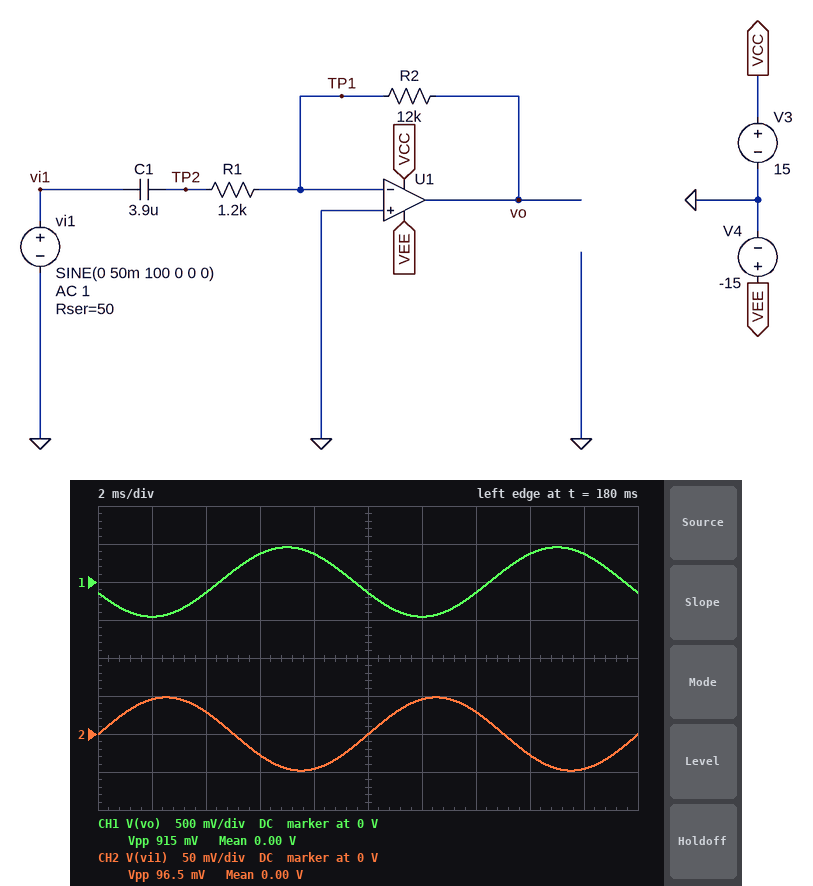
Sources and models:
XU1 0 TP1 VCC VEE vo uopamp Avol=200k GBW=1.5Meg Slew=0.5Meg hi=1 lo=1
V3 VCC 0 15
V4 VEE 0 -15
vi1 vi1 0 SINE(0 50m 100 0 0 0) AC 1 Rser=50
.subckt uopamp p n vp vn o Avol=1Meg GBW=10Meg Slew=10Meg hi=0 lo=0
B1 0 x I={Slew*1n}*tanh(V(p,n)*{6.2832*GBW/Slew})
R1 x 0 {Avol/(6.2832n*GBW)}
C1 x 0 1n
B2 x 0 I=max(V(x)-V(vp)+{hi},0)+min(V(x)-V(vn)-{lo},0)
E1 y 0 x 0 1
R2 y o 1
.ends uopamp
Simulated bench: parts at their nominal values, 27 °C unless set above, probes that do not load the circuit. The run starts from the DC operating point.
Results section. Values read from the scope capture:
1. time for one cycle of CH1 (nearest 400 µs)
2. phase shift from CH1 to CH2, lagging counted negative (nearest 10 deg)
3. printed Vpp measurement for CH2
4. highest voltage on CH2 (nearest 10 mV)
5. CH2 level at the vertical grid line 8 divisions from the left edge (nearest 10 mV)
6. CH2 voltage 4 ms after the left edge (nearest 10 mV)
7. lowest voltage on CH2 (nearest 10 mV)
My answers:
10.0 ms
160 deg
96.5 mV
50 mV
-30 mV
30 mV
-50 mV
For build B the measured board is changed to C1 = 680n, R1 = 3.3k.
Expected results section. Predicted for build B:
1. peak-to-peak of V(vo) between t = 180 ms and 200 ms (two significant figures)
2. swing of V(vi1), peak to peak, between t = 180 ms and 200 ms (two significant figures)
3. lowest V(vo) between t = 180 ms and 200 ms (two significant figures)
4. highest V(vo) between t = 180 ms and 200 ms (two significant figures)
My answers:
290 mV
99 mV
-150 mV
150 mV
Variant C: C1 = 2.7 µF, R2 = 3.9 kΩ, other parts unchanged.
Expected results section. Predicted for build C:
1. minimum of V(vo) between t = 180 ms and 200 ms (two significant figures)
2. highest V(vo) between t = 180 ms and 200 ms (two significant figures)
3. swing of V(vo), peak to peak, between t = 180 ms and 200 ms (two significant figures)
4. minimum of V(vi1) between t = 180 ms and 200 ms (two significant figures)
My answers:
-140 mV
140 mV
280 mV
-48 mV
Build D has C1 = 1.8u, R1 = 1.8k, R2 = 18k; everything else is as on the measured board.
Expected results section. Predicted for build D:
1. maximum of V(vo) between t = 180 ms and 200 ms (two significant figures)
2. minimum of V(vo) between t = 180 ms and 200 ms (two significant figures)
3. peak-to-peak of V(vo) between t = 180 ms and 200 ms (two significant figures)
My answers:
440 mV
-440 mV
880 mV
